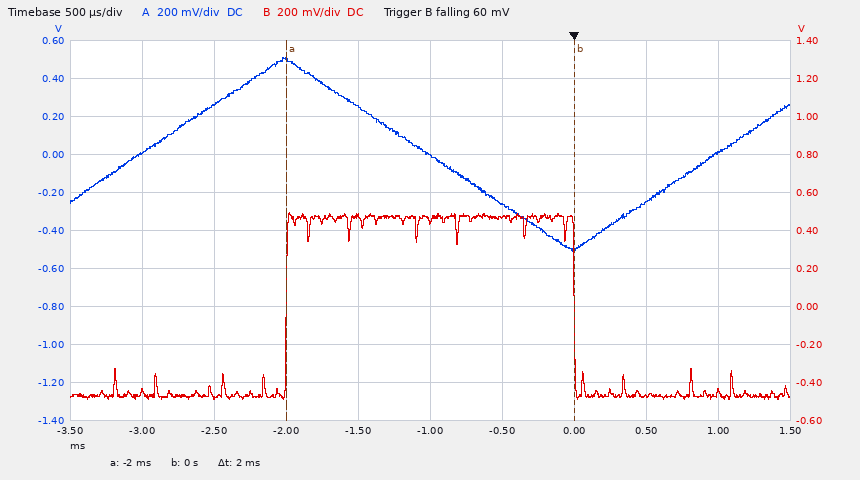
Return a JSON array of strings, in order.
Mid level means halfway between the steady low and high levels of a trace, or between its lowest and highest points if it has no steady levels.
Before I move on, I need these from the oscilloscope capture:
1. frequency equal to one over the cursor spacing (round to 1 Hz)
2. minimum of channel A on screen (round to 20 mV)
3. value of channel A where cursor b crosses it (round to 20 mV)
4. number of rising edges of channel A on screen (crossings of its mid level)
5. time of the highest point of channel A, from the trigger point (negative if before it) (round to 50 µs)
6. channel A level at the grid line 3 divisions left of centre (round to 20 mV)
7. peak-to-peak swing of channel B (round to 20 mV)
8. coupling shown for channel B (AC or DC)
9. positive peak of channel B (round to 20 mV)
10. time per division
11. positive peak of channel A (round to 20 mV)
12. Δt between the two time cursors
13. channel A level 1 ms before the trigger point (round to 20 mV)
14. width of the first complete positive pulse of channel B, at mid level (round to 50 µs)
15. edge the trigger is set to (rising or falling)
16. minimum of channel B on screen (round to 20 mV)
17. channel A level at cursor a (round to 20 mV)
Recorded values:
["500 Hz", "-520 mV", "-500 mV", "2", "-2.00 ms", "260 mV", "980 mV", "DC", "500 mV", "500 µs", "520 mV", "2 ms", "0 mV", "2.00 ms", "falling", "-480 mV", "500 mV"]
